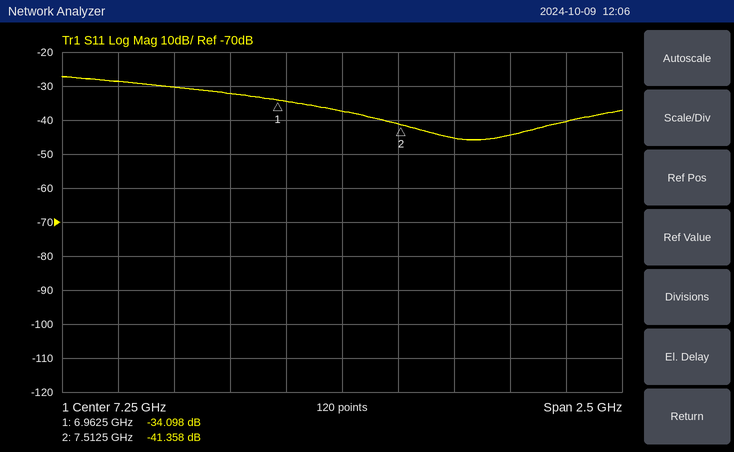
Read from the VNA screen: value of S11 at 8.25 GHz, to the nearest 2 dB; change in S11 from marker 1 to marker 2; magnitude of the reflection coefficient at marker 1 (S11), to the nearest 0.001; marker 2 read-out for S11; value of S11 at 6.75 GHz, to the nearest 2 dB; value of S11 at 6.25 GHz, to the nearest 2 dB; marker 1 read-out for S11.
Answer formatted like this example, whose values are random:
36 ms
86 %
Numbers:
-40 dB
-7.260 dB
0.020
-41.358 dB
-32 dB
-28 dB
-34.098 dB
